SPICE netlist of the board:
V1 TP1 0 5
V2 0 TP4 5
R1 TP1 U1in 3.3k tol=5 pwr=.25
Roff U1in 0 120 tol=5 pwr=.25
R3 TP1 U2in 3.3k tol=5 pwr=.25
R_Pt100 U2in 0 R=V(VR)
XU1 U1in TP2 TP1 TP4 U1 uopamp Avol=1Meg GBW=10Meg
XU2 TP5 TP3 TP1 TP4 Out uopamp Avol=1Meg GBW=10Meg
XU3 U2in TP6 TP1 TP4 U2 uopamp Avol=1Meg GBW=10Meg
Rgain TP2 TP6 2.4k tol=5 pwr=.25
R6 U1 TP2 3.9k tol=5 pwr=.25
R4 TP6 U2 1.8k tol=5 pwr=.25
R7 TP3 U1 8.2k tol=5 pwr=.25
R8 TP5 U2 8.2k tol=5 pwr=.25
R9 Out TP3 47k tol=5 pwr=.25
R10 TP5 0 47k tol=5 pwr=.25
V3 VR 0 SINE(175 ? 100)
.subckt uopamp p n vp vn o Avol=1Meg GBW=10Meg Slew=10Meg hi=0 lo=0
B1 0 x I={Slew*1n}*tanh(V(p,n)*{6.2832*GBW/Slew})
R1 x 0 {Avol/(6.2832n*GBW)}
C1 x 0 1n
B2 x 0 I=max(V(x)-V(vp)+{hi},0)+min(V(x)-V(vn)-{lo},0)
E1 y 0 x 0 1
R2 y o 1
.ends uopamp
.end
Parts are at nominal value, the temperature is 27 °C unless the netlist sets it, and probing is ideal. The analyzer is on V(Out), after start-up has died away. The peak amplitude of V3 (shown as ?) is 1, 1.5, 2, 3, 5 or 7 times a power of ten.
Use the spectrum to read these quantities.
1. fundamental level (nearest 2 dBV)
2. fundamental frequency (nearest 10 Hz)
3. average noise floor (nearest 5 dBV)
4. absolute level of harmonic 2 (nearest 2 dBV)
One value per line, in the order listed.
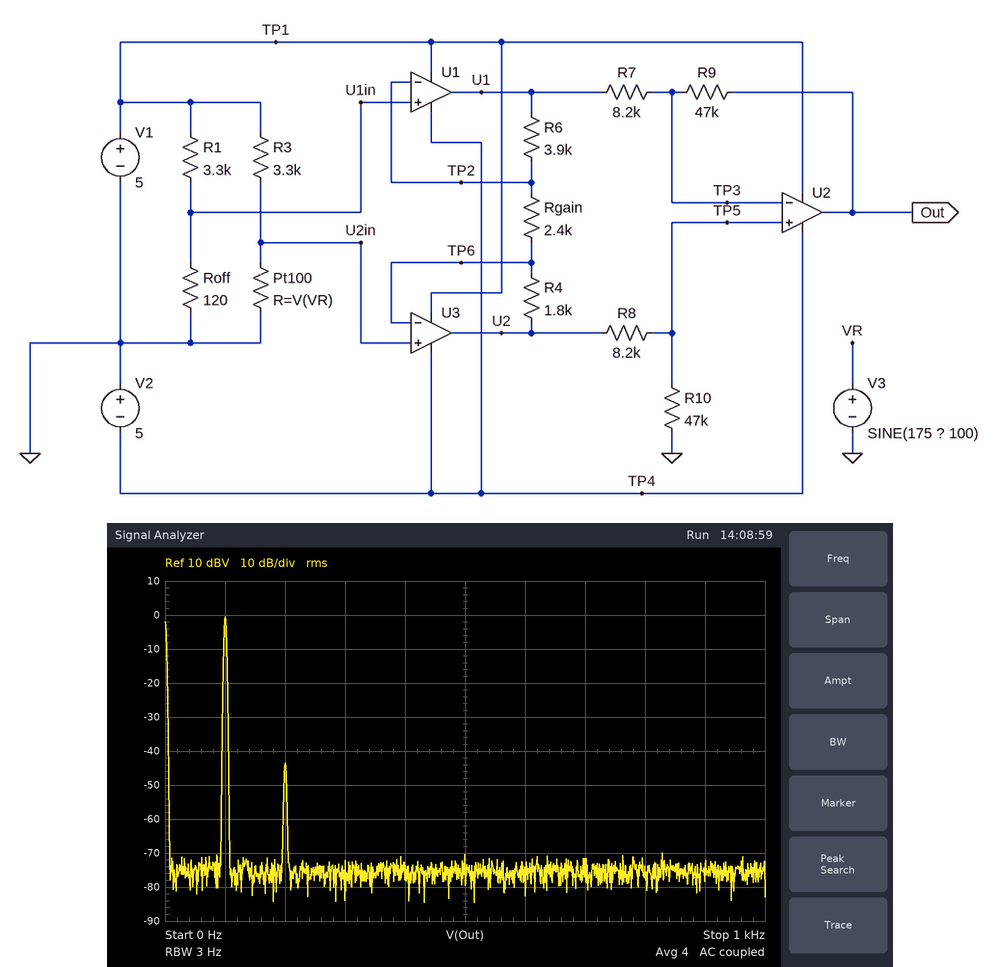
0 dBV
100 Hz
-75 dBV
-44 dBV
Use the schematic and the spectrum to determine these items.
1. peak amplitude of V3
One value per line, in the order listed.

50 V
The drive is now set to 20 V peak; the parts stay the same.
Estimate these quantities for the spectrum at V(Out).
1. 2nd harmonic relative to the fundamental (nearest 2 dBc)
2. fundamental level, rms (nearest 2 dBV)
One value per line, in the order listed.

-50 dBc
-8 dBV
